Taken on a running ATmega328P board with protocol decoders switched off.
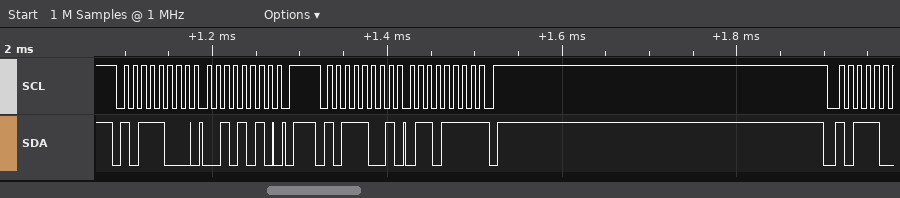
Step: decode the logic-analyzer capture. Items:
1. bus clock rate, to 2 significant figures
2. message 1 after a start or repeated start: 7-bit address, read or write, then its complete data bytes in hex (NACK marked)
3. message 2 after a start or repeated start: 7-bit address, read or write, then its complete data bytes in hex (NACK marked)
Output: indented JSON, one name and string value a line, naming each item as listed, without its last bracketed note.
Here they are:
{
  "bus clock rate, to 2 significant figures": "100 kHz",
  "message 1 after a start or repeated start: 7-bit address, read or write, then its complete data bytes in hex": "0x5C write: 2A",
  "message 2 after a start or repeated start: 7-bit address, read or write, then its complete data bytes in hex": "0x5C read: 6F NACK"
}
